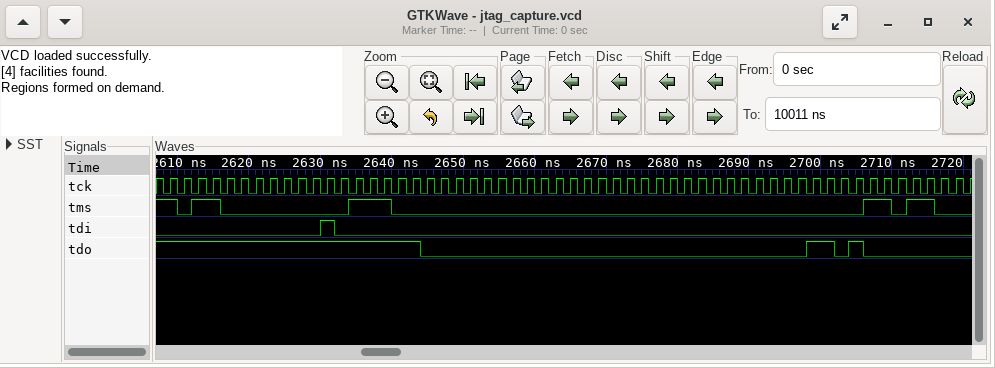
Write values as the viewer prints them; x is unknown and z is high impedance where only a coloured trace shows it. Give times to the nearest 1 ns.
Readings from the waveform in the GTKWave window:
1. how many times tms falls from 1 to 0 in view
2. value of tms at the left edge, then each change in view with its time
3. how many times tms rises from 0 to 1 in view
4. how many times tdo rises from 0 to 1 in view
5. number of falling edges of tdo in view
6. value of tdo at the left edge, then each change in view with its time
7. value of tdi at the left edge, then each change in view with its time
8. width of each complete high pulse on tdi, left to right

5
1, 0 at 2610 ns, 1 at 2612 ns, 0 at 2616 ns, 1 at 2634 ns, 0 at 2640 ns, 1 at 2706 ns, 0 at 2710 ns, 1 at 2712 ns, 0 at 2716 ns
4
2
3
1, 0 at 2644 ns, 1 at 2698 ns, 0 at 2702 ns, 1 at 2704 ns, 0 at 2706 ns
0, 1 at 2630 ns, 0 at 2632 ns
2 ns
